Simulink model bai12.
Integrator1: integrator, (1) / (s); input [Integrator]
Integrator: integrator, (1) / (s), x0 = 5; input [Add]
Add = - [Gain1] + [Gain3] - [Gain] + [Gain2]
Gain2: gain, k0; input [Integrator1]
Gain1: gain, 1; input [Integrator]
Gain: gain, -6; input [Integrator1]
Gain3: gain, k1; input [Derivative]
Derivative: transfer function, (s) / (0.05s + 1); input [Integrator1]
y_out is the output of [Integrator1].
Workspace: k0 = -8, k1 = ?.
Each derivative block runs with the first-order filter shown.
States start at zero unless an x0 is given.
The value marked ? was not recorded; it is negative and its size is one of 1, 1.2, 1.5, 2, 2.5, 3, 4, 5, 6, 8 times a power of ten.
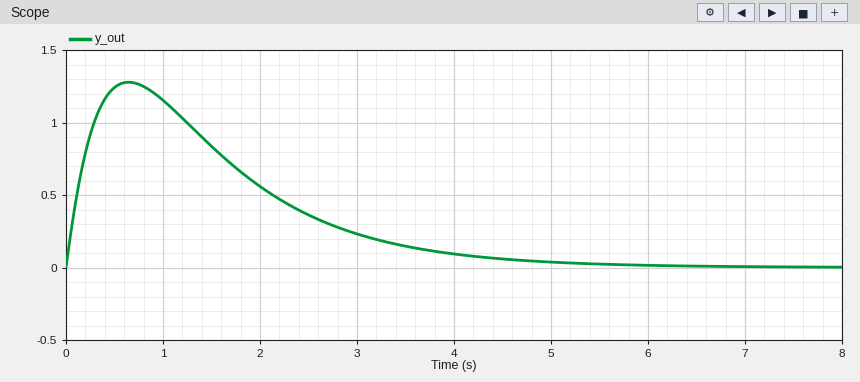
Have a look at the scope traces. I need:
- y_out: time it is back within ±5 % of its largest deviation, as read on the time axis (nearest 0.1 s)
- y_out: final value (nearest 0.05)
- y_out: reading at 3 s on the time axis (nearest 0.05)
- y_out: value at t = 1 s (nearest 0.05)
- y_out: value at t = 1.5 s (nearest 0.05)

4.4 s
0.00
0.25
1.15
0.85
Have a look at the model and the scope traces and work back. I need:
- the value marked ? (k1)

-2
